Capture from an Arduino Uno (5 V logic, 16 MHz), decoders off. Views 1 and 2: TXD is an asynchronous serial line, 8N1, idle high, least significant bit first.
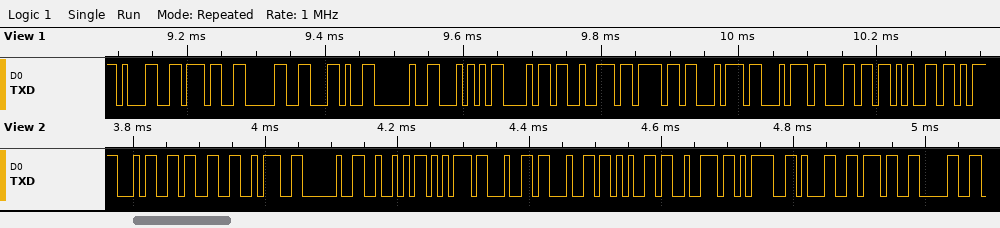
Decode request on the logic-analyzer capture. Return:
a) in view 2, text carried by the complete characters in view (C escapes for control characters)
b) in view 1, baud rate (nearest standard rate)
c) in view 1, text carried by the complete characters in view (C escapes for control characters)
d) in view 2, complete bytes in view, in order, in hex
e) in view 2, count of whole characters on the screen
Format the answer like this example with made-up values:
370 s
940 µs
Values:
"43: Rudder=170"
115200 baud
"170, Throttle"
34 33 3A 20 52 75 64 64 65 72 3D 31 37 30
14
